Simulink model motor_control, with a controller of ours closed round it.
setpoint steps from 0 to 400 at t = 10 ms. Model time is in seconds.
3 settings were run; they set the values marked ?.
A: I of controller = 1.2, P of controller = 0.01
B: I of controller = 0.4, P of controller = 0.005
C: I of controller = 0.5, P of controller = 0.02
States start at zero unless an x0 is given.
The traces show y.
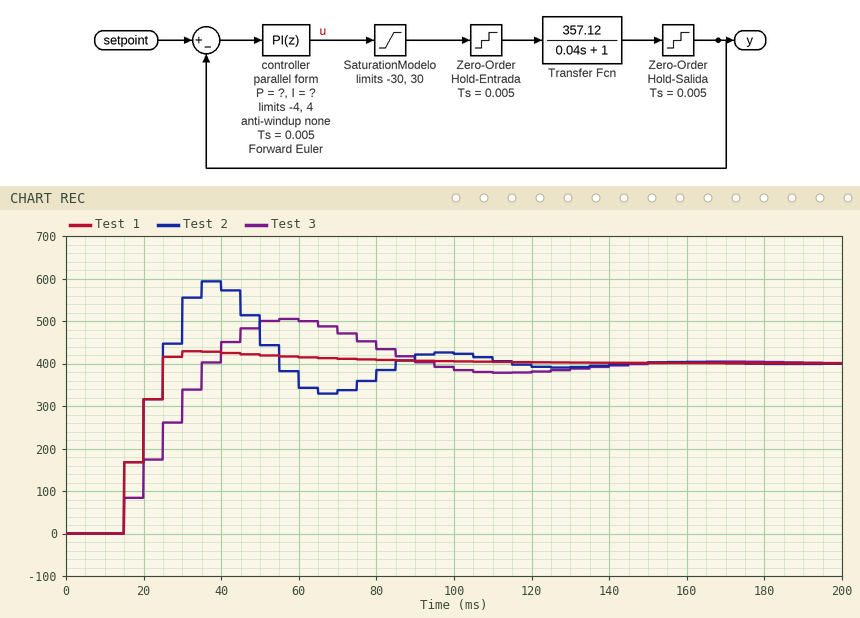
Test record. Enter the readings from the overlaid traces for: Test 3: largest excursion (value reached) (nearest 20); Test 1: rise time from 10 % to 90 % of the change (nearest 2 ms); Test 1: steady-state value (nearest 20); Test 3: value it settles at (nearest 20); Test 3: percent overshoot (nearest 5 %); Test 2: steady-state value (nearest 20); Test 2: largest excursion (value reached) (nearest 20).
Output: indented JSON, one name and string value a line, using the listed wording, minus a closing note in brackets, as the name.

{
  "Test 3: largest excursion (value reached)": "500",
  "Test 1: rise time from 10 % to 90 % of the change": "10 ms",
  "Test 1: steady-state value": "400",
  "Test 3: value it settles at": "400",
  "Test 3: percent overshoot": "25 %",
  "Test 2: steady-state value": "400",
  "Test 2: largest excursion (value reached)": "600"
}
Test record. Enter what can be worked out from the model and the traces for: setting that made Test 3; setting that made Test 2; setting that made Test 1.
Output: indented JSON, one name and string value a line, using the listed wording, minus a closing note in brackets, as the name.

{
  "setting that made Test 3": "B",
  "setting that made Test 2": "A",
  "setting that made Test 1": "C"
}
